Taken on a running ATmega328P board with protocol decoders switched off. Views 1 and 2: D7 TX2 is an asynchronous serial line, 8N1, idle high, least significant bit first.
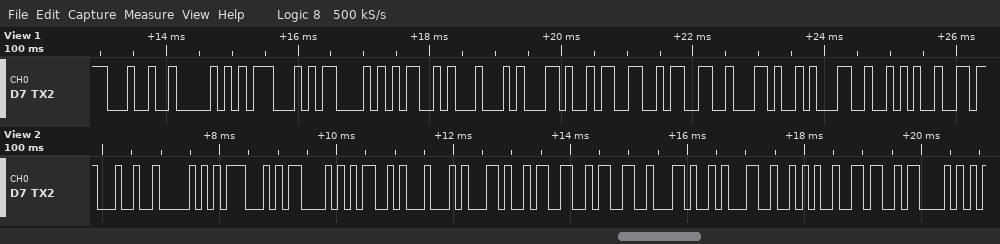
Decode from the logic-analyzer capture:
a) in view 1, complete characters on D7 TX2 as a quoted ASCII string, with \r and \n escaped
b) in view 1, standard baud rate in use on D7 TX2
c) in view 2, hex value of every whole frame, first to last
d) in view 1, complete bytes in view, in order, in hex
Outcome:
"$PGCMD,33,1*"
9600 baud
0x24 0x50 0x47 0x43 0x4D 0x44 0x2C 0x33 0x33 0x2C 0x31 0x2A 0x36 0x43
0x24 0x50 0x47 0x43 0x4D 0x44 0x2C 0x33 0x33 0x2C 0x31 0x2A
